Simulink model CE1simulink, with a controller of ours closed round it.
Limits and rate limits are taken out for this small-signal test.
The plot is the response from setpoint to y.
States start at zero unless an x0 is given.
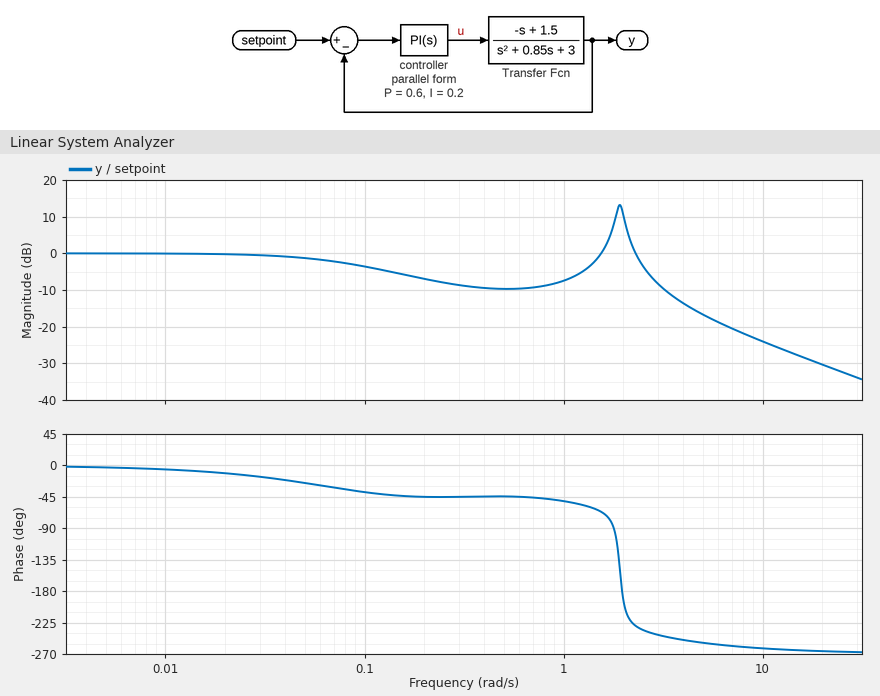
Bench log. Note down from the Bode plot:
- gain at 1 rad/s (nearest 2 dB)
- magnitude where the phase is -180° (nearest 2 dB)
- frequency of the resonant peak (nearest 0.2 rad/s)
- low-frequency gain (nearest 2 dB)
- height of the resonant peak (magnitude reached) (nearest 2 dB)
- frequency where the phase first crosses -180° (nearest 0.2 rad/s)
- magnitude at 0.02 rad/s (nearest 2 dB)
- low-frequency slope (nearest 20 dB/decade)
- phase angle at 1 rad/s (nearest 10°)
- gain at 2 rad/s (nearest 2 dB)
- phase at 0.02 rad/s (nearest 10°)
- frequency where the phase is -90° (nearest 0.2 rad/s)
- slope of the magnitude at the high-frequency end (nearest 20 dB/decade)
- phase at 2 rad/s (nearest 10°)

-8 dB
12 dB
2.0 rad/s
0 dB
14 dB
2.0 rad/s
0 dB
0 dB/decade
-50°
10 dB
-10°
1.8 rad/s
-20 dB/decade
-190°
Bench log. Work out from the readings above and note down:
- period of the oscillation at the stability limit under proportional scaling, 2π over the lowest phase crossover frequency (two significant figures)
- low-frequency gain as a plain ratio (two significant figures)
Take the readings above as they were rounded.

3.1 s
1.0
